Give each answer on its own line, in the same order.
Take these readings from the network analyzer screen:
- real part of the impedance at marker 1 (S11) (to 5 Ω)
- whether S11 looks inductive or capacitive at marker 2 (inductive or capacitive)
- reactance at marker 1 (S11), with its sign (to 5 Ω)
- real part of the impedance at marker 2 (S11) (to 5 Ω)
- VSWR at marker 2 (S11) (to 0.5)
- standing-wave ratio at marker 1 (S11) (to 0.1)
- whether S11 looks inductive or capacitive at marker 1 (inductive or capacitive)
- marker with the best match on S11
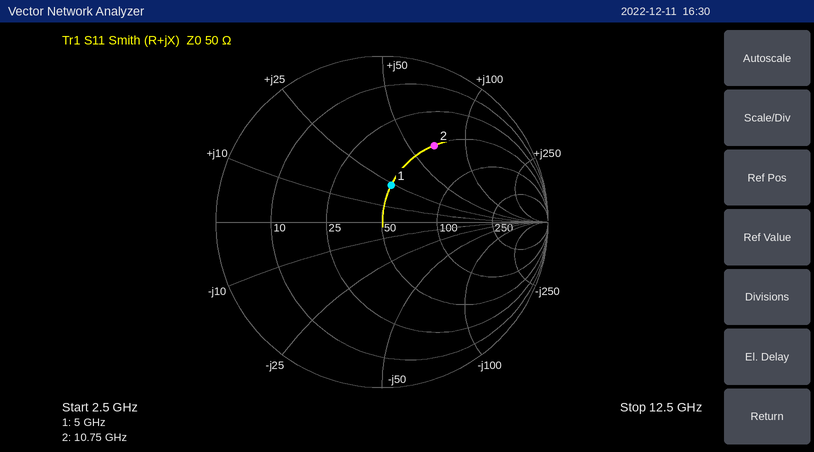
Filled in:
50 Ω
inductive
+25 Ω
50 Ω
3.5
1.6
inductive
marker 1
